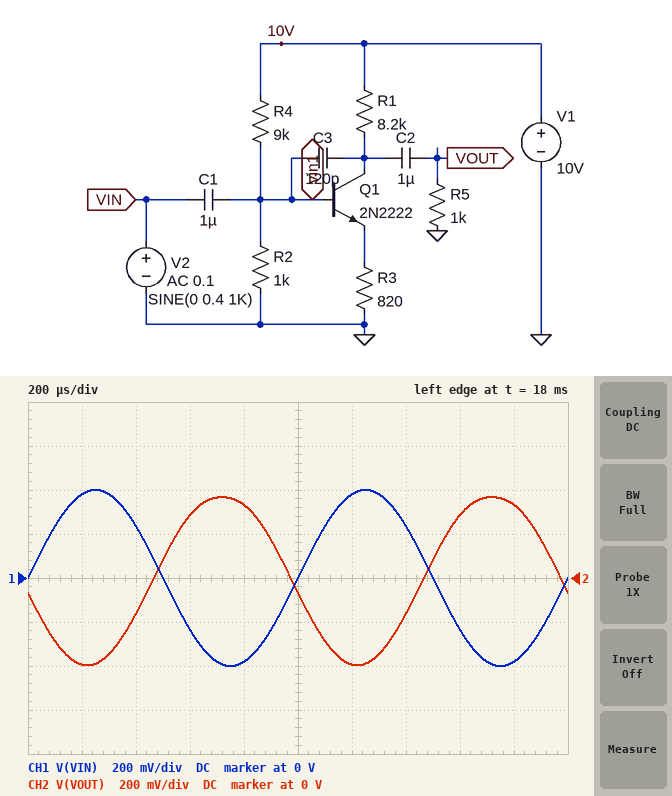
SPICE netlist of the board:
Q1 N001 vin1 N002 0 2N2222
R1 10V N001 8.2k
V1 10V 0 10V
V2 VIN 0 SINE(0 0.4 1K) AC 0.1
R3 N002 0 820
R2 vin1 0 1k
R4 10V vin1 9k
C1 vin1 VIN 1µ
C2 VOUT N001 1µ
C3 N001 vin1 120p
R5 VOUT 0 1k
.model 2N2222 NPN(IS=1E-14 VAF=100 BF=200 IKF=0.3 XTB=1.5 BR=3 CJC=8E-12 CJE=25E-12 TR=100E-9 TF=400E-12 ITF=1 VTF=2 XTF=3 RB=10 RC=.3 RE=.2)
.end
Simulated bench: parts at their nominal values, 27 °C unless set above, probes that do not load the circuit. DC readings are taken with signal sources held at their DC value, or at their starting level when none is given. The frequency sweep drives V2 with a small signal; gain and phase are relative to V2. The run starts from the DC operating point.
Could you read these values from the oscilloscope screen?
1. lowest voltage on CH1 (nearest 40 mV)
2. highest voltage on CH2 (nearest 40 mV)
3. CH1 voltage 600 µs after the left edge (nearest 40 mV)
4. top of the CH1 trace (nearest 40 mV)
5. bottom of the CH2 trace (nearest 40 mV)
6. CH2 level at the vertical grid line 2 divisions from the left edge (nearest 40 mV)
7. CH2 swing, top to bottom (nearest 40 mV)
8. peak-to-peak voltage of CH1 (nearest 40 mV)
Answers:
-400 mV
360 mV
-240 mV
400 mV
-400 mV
-160 mV
760 mV
800 mV
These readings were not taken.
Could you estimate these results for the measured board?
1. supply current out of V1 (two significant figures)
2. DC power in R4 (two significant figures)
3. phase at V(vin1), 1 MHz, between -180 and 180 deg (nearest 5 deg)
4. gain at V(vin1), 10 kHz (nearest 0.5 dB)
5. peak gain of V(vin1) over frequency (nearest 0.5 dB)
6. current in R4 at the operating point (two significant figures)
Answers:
1.4 mA
9.0 mW
0 deg
0 dB
0 dB
1.0 mA
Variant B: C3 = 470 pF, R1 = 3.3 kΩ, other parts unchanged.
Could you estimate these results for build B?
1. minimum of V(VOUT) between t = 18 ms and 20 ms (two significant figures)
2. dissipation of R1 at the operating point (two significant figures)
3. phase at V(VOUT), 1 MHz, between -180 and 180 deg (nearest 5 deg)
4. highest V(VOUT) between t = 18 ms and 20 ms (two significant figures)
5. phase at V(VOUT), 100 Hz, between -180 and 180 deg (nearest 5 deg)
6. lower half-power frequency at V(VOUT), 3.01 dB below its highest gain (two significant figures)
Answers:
-340 mV
650 µW
45 deg
320 mV
-100 deg
260 Hz
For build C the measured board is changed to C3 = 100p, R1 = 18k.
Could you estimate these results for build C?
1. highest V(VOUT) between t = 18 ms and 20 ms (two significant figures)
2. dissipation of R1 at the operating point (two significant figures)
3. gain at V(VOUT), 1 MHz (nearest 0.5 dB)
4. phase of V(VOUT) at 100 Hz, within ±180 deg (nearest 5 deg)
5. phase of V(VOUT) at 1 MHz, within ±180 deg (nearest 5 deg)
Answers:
390 mV
3.5 mW
0.5 dB
-115 deg
115 deg
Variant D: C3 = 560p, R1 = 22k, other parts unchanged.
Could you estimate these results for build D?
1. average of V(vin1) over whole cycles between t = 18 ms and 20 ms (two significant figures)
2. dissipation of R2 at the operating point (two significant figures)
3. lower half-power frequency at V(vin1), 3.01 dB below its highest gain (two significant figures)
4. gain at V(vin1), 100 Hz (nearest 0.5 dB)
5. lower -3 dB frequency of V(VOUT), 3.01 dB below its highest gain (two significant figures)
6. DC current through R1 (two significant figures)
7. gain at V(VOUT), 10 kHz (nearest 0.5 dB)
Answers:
980 mV
990 µW
210 Hz
-7.5 dB
390 Hz
430 µA
-2.0 dB
